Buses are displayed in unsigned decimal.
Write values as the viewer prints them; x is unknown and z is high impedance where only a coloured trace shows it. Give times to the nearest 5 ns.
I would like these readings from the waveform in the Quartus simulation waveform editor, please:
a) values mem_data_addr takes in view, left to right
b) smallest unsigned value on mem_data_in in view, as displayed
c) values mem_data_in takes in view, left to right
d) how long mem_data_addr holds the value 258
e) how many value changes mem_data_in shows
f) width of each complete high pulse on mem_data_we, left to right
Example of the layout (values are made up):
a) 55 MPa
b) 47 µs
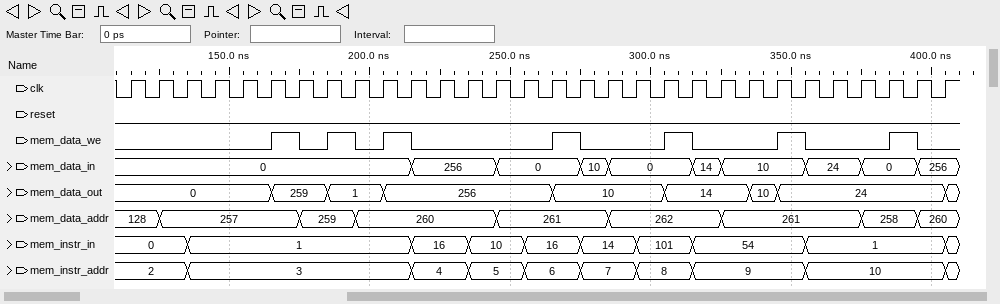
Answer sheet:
a) 128, 257, 259, 260, 261, 262, 261, 258, 260
b) 0
c) 0, 256, 0, 10, 0, 14, 10, 24, 0, 256
d) 20 ns
e) 9
f) 10 ns, 10 ns, 10 ns, 10 ns, 10 ns, 10 ns, 10 ns
